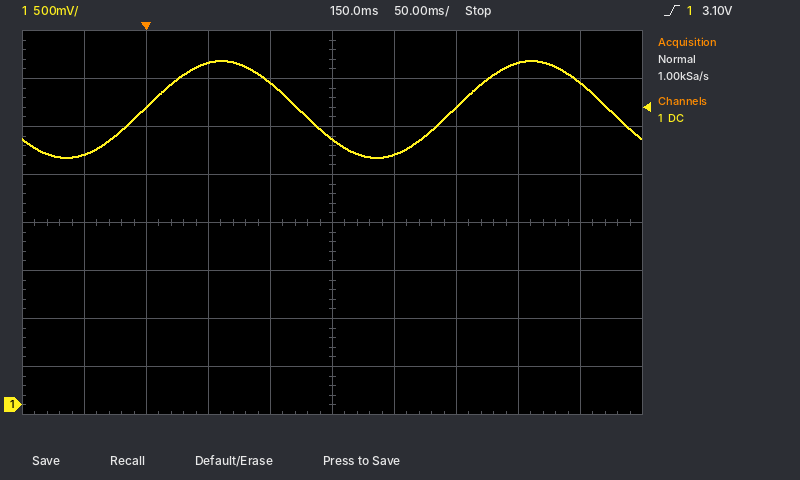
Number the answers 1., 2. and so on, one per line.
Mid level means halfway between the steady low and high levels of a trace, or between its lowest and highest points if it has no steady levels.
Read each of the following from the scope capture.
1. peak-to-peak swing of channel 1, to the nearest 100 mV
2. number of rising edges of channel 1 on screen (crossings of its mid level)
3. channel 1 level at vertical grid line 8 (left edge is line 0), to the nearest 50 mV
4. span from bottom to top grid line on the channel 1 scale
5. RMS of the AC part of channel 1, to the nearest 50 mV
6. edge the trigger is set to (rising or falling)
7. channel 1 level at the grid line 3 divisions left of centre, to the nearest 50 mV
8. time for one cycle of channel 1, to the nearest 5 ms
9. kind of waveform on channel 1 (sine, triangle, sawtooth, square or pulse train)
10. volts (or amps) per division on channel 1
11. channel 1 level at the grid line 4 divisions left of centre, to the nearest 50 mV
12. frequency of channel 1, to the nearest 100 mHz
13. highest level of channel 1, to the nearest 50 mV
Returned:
1. 1.00 V
2. 2
3. 3.55 V
4. 4 V
5. 350 mV
6. rising
7. 3.10 V
8. 250 ms
9. sine
10. 500 mV
11. 2.60 V
12. 4.0 Hz
13. 3.60 V
